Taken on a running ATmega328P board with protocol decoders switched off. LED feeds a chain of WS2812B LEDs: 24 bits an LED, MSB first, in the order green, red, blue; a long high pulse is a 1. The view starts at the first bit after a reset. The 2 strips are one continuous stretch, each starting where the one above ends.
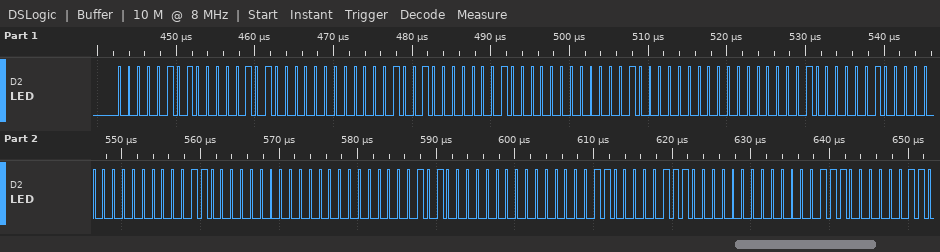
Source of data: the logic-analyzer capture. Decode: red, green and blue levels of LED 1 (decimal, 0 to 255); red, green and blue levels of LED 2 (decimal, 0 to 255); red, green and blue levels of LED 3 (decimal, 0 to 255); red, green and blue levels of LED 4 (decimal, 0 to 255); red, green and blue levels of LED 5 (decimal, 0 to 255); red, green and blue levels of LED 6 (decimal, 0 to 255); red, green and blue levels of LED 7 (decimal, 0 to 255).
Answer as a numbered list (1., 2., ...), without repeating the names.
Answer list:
1. 5, 5, 0
2. 1, 9, 0
3. 0, 8, 2
4. 0, 4, 6
5. 0, 0, 10
6. 3, 0, 7
7. 7, 0, 3
